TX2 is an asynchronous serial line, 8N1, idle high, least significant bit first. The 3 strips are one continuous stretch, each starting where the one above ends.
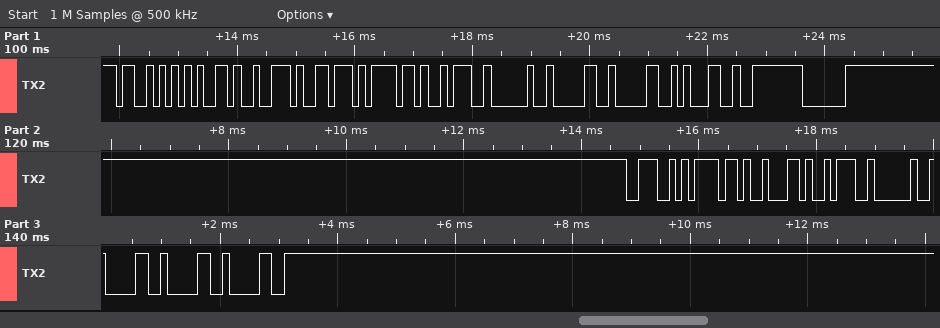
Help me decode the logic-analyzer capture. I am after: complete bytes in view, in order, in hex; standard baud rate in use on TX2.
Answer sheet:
53 65 72 76 6F 3A 20 30 30 31 FE C0 4E 6F 62 3A 20 30 30 30
9600 baud
